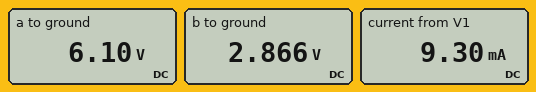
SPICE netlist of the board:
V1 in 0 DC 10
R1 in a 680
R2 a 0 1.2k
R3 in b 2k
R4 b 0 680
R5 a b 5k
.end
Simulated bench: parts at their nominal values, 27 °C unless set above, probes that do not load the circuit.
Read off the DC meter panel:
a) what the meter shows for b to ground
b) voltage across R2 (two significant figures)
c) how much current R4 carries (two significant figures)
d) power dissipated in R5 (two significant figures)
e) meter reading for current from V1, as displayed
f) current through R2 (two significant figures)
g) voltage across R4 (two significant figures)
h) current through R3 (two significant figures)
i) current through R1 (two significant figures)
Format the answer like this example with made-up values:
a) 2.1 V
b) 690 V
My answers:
a) 2.866 V
b) 6.1 V
c) 4.2 mA
d) 2.1 mW
e) 9.30 mA
f) 5.1 mA
g) 2.9 V
h) 3.6 mA
i) 5.7 mA
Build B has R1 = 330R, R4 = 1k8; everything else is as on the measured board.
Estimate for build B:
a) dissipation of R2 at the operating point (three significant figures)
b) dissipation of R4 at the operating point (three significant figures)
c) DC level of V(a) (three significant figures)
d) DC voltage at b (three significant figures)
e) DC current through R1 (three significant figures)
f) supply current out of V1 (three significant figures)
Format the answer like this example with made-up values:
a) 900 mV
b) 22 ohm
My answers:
a) 49.6 mW
b) 15.1 mW
c) 7.71 V
d) 5.21 V
e) 6.93 mA
f) 9.32 mA
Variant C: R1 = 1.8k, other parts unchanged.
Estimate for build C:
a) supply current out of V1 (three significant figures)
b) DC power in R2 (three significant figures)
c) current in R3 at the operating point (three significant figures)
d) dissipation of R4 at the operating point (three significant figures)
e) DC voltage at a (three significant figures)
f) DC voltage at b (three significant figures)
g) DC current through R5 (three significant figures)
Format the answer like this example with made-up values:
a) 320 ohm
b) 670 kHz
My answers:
a) 7.10 mA
b) 12.2 mW
c) 3.67 mA
d) 10.4 mW
e) 3.83 V
f) 2.66 V
g) 235 µA
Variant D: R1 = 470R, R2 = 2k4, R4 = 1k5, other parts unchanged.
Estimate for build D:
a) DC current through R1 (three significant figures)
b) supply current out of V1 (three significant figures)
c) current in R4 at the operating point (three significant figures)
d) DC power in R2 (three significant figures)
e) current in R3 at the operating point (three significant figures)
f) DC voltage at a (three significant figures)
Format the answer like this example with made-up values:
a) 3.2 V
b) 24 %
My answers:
a) 4.03 mA
b) 6.61 mA
c) 3.23 mA
d) 27.4 mW
e) 2.58 mA
f) 8.11 V
